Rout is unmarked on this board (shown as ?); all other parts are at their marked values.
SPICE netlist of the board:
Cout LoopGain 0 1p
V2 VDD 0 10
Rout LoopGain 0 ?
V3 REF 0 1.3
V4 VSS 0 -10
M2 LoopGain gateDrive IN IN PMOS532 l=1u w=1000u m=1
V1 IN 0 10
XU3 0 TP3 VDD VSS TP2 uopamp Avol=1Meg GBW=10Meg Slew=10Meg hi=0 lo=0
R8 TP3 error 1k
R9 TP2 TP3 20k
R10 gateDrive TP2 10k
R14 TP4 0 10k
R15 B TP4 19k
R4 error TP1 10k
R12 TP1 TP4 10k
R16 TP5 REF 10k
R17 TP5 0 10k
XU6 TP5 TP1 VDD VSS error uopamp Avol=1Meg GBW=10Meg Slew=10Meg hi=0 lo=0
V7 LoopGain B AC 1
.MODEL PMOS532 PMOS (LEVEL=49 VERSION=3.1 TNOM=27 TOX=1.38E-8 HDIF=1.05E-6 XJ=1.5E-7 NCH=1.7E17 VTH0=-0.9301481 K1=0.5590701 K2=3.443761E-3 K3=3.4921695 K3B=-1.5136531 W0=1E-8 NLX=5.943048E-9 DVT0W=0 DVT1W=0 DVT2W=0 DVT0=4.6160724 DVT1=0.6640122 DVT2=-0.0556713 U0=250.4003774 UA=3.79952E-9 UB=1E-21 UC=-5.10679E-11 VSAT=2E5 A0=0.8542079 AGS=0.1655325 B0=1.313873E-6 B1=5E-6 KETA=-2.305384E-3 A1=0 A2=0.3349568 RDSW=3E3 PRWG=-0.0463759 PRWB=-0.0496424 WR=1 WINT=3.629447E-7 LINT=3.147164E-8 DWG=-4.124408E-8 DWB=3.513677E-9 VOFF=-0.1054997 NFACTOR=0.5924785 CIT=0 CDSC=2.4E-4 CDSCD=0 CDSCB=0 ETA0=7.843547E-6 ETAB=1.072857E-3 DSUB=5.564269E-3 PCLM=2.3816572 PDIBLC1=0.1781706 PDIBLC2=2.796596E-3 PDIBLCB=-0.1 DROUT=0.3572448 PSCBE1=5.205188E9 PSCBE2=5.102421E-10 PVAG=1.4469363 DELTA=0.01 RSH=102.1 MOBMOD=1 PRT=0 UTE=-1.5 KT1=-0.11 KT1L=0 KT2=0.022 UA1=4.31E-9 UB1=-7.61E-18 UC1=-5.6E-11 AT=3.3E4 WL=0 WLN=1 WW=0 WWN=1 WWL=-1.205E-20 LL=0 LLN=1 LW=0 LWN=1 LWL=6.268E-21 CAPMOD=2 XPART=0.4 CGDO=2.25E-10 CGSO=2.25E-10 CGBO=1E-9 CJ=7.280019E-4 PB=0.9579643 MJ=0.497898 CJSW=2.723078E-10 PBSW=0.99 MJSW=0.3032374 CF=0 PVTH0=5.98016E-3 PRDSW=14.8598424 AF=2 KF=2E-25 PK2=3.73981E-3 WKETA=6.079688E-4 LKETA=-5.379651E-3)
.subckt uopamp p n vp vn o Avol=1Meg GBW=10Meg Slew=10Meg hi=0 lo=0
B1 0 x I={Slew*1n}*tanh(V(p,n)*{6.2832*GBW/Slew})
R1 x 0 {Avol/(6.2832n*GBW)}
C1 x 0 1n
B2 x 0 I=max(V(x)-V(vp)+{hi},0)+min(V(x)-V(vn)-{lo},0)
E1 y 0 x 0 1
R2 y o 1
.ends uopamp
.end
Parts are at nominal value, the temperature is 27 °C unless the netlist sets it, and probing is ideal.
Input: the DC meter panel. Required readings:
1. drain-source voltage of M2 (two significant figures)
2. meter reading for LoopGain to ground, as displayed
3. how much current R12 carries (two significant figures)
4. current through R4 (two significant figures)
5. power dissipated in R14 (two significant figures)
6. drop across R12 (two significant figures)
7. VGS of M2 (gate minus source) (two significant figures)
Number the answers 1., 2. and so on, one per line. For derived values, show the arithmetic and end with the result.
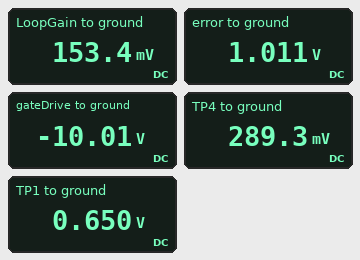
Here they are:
1. 153.4 mV - 10 V = -9.8 V
2. 153.4 mV
3. (650 mV - 289.3 mV) / 10 kΩ = 36 µA
4. (1.011 V - 650 mV) / 10 kΩ = 36 µA
5. (289.3 mV)^2 / 10 kΩ = 8.4 µW
6. 650 mV - 289.3 mV = 360 mV
7. -10.01 V - 10 V = -20 V
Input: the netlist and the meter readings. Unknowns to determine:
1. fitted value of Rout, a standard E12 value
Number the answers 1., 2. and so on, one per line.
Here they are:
1. 3.3 Ω
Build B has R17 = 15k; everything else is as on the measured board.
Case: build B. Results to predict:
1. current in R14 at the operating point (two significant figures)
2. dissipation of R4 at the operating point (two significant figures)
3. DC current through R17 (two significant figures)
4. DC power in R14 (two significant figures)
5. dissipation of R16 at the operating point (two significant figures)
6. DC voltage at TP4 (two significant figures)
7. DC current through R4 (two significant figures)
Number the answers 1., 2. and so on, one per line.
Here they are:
1. 34 µA
2. 19 µW
3. 52 µA
4. 12 µW
5. 27 µW
6. 340 mV
7. 44 µA
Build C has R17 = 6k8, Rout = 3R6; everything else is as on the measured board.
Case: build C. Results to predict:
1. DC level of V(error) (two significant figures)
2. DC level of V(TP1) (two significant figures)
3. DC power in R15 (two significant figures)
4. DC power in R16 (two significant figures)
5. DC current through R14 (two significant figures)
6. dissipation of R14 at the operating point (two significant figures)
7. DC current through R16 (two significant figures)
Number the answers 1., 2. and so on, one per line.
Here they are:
1. 810 mV
2. 530 mV
3. 300 nW
4. 60 µW
5. 24 µA
6. 5.9 µW
7. 77 µA
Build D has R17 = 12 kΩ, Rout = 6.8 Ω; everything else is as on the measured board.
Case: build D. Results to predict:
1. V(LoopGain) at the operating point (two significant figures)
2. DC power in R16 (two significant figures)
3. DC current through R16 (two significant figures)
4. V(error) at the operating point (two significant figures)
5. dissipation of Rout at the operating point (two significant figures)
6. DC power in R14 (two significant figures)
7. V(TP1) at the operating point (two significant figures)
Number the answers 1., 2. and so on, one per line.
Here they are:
1. 310 mV
2. 35 µW
3. 59 µA
4. 1.1 V
5. 14 mW
6. 12 µW
7. 710 mV
